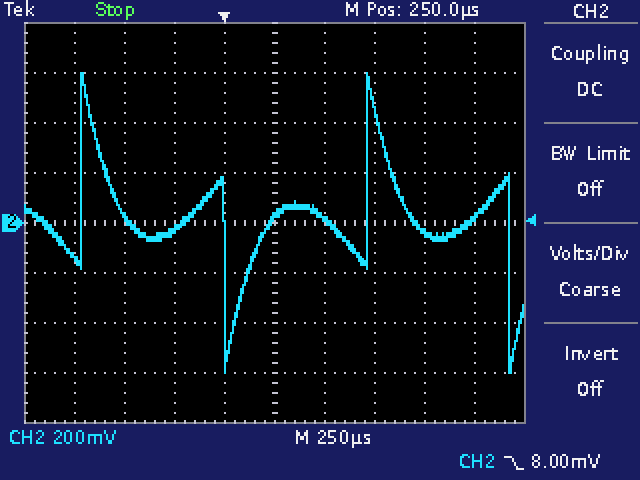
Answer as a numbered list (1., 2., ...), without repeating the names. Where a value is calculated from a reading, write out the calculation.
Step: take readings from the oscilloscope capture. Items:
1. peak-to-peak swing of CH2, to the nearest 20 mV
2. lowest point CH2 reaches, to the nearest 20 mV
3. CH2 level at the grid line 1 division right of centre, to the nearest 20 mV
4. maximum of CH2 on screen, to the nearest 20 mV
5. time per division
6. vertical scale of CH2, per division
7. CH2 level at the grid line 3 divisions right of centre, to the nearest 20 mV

1. 600 mV − (-600 mV) = 1.20 V
2. -600 mV
3. 20 mV
4. 600 mV
5. 250 µs
6. 200 mV
7. -40 mV
